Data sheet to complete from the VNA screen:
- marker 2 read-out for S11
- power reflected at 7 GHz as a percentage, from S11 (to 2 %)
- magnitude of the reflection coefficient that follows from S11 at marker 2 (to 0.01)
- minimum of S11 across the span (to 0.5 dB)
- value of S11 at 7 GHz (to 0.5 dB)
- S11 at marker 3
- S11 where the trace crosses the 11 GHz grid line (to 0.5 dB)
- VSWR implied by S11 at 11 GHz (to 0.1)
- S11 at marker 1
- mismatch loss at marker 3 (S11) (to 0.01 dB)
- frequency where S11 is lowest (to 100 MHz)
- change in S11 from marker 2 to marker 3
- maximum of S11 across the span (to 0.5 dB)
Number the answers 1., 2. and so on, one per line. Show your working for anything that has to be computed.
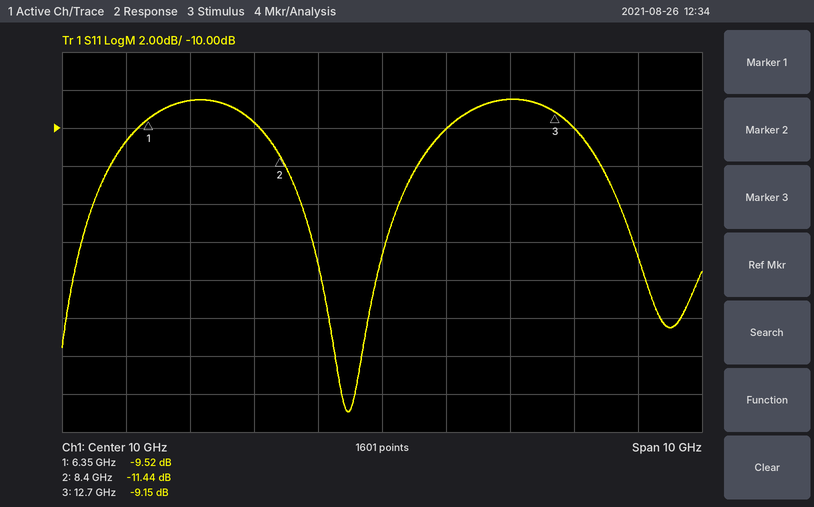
1. -11.44 dB
2. 10^(-8.5/10) ≈ 14 %
3. 10^(-11.44/20) ≈ 0.27
4. -25.0 dB
5. -8.5 dB
6. -9.15 dB
7. -10.0 dB
8. |Γ| = 10^(-10/20) = 0.3162; VSWR = (1 + 0.3162)/(1 − 0.3162) ≈ 1.9
9. -9.52 dB
10. −10 log10(1 − 10^(-9.15/10)) ≈ 0.56 dB
11. 9.5 GHz
12. -9.15 − (-11.44) = 2.29 dB
13. -8.5 dB
